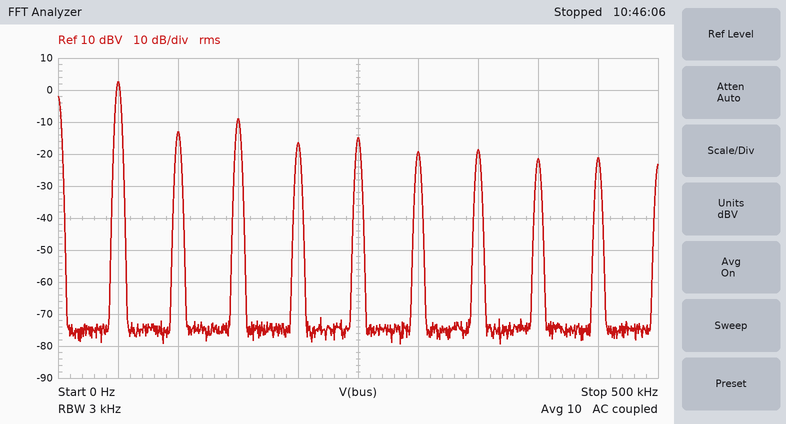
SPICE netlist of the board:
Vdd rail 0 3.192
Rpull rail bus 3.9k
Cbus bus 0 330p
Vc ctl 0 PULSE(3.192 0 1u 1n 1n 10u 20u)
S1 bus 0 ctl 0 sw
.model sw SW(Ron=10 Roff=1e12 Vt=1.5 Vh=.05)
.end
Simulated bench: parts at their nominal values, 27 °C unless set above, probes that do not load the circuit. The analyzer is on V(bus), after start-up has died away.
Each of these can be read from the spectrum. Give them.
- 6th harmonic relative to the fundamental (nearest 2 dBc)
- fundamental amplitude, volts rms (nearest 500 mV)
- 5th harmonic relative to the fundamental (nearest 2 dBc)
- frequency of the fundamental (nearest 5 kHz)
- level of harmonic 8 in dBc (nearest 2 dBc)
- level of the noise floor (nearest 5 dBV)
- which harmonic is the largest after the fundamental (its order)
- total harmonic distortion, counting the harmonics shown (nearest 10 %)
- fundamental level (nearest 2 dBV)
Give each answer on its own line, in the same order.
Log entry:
-22 dBc
1.5 V
-18 dBc
50 kHz
-24 dBc
-75 dBV
3
40 %
2 dBV
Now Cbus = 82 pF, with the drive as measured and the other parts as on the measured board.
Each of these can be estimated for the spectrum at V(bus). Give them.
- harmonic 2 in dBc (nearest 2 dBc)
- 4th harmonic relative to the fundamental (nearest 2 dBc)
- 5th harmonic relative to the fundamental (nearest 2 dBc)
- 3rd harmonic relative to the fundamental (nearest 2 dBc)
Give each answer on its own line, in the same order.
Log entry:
-26 dBc
-26 dBc
-14 dBc
-10 dBc
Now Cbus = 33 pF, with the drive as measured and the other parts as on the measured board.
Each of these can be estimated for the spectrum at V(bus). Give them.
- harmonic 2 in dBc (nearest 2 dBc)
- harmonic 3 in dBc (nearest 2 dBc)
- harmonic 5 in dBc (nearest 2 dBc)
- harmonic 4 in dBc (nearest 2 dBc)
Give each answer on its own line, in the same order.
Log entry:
-34 dBc
-10 dBc
-14 dBc
-34 dBc
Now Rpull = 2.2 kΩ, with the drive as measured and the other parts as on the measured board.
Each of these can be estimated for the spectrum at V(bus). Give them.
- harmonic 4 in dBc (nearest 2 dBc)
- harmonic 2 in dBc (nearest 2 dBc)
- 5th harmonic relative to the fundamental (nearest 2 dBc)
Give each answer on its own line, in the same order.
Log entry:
-22 dBc
-20 dBc
-16 dBc
